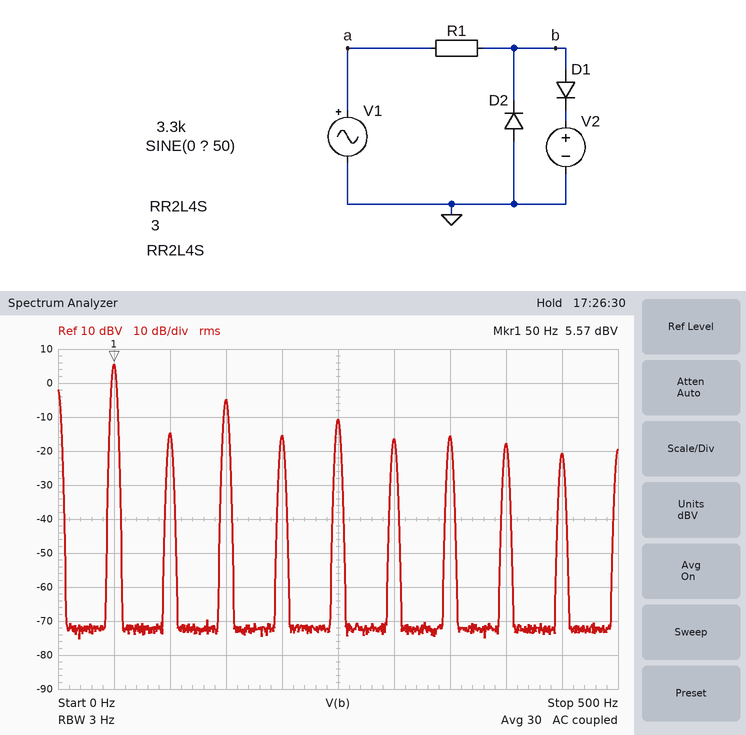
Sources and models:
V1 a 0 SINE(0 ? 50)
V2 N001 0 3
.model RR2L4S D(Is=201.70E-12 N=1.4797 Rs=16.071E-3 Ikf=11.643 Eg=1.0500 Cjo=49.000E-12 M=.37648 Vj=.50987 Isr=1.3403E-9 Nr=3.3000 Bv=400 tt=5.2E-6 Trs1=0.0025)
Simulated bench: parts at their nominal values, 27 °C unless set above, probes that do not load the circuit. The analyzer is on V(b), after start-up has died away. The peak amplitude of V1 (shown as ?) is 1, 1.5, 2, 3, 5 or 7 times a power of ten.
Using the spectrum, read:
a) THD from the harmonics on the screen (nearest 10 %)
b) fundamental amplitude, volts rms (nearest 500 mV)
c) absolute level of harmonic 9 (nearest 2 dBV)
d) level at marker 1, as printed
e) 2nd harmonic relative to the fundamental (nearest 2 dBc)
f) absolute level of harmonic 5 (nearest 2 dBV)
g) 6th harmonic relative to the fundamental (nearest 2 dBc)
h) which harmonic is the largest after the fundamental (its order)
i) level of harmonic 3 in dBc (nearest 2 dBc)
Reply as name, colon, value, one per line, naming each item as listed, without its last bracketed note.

THD from the harmonics on the screen: 40 %
fundamental amplitude, volts rms: 2.0 V
absolute level of harmonic 9: -20 dBV
level at marker 1, as printed: 5.57 dBV
2nd harmonic relative to the fundamental: -20 dBc
absolute level of harmonic 5: -10 dBV
6th harmonic relative to the fundamental: -22 dBc
which harmonic is the largest after the fundamental: 3
level of harmonic 3 in dBc: -10 dBc
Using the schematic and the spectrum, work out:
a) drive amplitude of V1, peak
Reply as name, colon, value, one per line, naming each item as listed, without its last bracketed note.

drive amplitude of V1, peak: 15 V
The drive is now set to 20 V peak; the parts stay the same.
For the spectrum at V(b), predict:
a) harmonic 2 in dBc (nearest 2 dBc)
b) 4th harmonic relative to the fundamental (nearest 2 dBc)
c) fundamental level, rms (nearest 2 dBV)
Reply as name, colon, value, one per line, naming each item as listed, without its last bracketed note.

harmonic 2 in dBc: -22 dBc
4th harmonic relative to the fundamental: -24 dBc
fundamental level, rms: 6 dBV
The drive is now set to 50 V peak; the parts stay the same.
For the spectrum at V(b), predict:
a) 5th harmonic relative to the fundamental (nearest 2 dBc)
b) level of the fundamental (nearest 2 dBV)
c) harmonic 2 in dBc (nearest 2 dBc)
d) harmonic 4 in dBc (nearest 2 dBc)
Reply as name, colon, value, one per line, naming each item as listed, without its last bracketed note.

5th harmonic relative to the fundamental: -14 dBc
level of the fundamental: 6 dBV
harmonic 2 in dBc: -30 dBc
harmonic 4 in dBc: -30 dBc
